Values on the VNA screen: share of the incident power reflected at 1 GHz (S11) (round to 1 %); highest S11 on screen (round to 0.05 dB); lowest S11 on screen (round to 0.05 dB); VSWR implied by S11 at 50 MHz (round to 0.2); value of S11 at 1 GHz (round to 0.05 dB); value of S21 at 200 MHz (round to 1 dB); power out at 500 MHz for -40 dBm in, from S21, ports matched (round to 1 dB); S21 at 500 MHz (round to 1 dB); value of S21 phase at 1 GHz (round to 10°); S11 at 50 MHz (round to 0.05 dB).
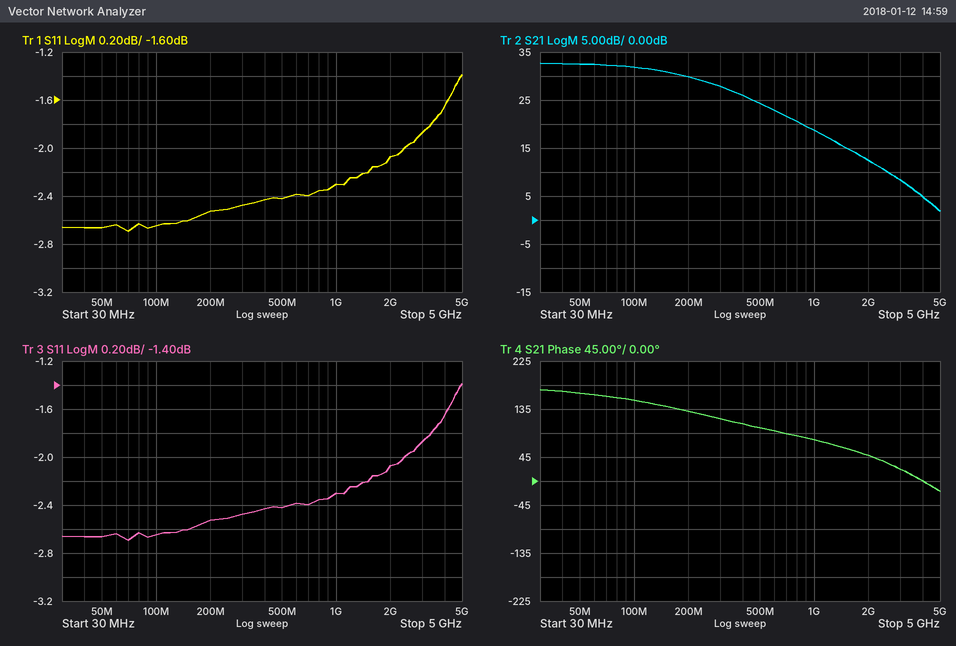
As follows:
59 %
-1.40 dB
-2.70 dB
6.6
-2.30 dB
30 dB
-16 dBm
24 dB
80°
-2.65 dB
